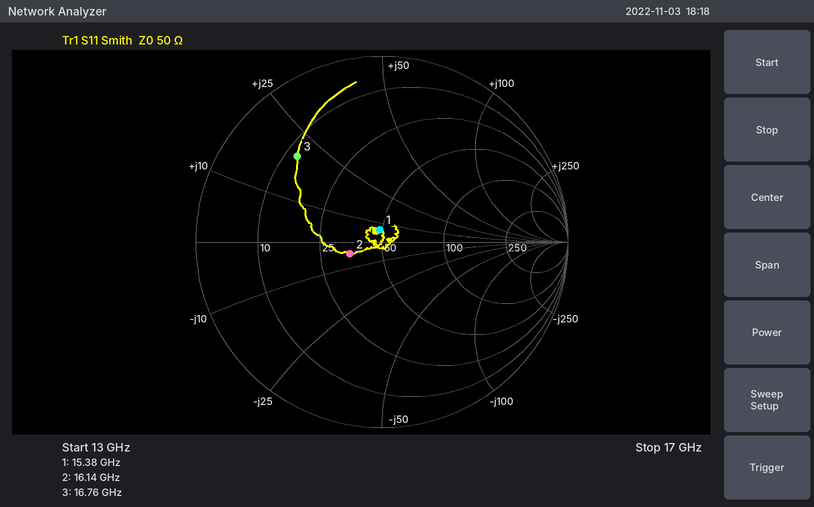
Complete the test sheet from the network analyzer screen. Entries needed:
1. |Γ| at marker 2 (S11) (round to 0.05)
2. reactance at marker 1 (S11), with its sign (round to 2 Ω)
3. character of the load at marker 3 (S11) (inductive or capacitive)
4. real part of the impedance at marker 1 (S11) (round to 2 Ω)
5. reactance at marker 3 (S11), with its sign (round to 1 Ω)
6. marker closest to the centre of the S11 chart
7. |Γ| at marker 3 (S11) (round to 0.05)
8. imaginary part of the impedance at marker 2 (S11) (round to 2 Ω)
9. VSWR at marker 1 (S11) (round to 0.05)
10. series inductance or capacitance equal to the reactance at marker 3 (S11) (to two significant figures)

0.20
+6 Ω
inductive
48 Ω
+20 Ω
marker 1
0.65
-4 Ω
1.15
190 pH
